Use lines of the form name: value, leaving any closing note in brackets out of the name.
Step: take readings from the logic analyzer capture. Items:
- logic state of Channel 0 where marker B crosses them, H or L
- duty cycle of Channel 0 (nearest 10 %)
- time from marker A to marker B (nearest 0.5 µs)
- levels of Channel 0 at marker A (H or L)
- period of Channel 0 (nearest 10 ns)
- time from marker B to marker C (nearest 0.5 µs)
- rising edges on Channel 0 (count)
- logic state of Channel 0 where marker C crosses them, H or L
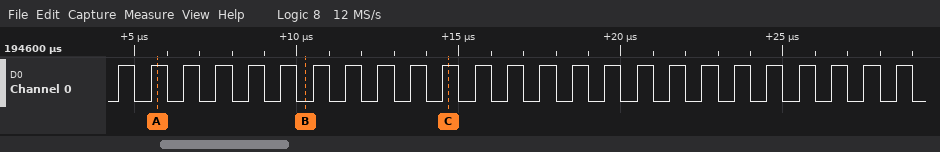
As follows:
logic state of Channel 0 where marker B crosses them, H or L: Channel 0=L
duty cycle of Channel 0: 50 %
time from marker A to marker B: 4.5 µs
levels of Channel 0 at marker A: Channel 0=H
period of Channel 0: 1000 ns
time from marker B to marker C: 4.5 µs
rising edges on Channel 0: 25
logic state of Channel 0 where marker C crosses them, H or L: Channel 0=H
